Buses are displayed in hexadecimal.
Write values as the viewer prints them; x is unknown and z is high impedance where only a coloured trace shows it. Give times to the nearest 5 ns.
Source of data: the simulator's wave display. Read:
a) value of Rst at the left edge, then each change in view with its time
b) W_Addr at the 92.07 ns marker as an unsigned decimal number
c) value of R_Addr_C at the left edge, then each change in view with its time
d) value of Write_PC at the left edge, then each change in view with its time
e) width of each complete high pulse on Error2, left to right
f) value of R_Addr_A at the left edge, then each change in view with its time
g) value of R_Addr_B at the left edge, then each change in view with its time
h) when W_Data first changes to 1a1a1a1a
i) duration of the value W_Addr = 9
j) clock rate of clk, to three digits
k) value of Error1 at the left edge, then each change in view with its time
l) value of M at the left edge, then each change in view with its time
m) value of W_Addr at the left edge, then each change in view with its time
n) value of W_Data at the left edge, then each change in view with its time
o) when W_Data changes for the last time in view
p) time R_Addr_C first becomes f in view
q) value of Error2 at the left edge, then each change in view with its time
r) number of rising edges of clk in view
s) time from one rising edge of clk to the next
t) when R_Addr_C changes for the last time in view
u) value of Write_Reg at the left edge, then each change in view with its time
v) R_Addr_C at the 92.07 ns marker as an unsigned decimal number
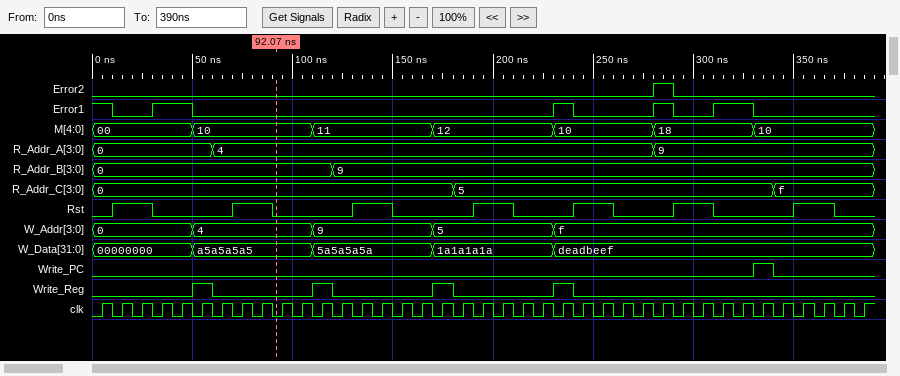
0, 1 at 10 ns, 0 at 30 ns, 1 at 70 ns, 0 at 90 ns, 1 at 130 ns, 0 at 150 ns, 1 at 190 ns, 0 at 210 ns, 1 at 240 ns, 0 at 260 ns, 1 at 290 ns, 0 at 310 ns, 1 at 350 ns, 0 at 370 ns
4
0, 5 at 180 ns, f at 340 ns
0, 1 at 330 ns, 0 at 340 ns
10 ns
0, 4 at 60 ns, 9 at 280 ns
0, 9 at 120 ns
170 ns
60 ns
100 MHz
1, 0 at 10 ns, 1 at 30 ns, 0 at 50 ns, 1 at 230 ns, 0 at 240 ns, 1 at 280 ns, 0 at 290 ns, 1 at 310 ns, 0 at 330 ns
00, 10 at 50 ns, 11 at 110 ns, 12 at 170 ns, 10 at 230 ns, 18 at 280 ns, 10 at 330 ns
0, 4 at 50 ns, 9 at 110 ns, 5 at 170 ns, f at 230 ns
00000000, a5a5a5a5 at 50 ns, 5a5a5a5a at 110 ns, 1a1a1a1a at 170 ns, deadbeef at 230 ns
230 ns
340 ns
0, 1 at 280 ns, 0 at 290 ns
39
10 ns
340 ns
0, 1 at 50 ns, 0 at 60 ns, 1 at 110 ns, 0 at 120 ns, 1 at 170 ns, 0 at 180 ns, 1 at 230 ns, 0 at 240 ns
0
